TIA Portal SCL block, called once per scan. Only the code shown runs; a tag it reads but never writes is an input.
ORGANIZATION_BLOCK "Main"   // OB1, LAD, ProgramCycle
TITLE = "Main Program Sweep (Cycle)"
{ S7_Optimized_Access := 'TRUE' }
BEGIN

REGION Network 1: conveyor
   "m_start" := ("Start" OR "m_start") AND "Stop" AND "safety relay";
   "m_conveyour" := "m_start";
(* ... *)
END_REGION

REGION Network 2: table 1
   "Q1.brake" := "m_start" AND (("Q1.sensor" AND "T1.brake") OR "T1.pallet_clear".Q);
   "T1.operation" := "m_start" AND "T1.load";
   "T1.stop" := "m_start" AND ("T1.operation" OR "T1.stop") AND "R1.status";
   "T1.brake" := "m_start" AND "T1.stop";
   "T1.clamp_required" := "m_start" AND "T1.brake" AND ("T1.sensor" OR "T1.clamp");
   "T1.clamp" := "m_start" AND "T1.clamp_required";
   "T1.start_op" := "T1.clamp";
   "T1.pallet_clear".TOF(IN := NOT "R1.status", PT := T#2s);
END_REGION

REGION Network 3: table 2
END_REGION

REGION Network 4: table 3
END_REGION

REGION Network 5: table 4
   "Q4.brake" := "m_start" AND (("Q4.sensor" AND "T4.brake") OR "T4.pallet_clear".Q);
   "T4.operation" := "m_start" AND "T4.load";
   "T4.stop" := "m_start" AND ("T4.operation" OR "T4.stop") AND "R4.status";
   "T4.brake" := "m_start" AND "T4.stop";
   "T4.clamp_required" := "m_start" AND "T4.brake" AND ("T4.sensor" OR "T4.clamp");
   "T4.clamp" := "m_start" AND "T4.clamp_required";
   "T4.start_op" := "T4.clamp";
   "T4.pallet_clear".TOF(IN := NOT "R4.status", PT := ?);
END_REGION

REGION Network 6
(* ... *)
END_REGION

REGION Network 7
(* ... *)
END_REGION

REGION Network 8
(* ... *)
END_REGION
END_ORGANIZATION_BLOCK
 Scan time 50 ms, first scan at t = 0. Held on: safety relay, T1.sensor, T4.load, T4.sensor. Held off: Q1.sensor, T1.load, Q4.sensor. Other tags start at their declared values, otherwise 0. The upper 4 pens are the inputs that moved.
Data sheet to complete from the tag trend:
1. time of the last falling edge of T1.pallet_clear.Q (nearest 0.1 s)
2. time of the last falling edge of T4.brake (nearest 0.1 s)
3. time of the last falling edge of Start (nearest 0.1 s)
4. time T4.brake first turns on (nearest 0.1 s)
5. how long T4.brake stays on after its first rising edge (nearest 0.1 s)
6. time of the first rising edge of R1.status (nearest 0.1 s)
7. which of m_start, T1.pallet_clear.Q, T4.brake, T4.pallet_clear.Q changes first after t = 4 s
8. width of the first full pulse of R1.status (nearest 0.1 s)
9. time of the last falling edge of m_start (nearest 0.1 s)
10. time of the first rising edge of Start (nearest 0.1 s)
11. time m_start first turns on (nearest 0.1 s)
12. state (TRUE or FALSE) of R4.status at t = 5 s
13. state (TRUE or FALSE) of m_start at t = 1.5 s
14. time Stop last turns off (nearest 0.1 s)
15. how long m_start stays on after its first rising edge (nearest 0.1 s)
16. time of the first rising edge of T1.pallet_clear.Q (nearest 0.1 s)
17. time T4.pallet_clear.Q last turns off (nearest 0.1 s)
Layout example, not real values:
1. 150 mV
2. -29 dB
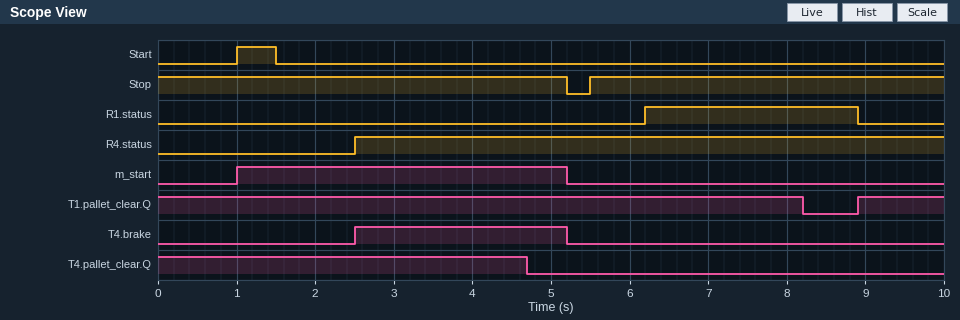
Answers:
1. 8.2 s
2. 5.2 s
3. 1.5 s
4. 2.5 s
5. 2.7 s
6. 6.2 s
7. T4.pallet_clear.Q
8. 2.7 s
9. 5.2 s
10. 1.0 s
11. 1.0 s
12. TRUE
13. TRUE
14. 5.2 s
15. 4.2 s
16. 8.9 s
17. 4.7 s
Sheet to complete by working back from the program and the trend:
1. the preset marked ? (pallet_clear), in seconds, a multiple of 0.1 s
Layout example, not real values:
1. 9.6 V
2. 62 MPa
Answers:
1. 2.2 s
